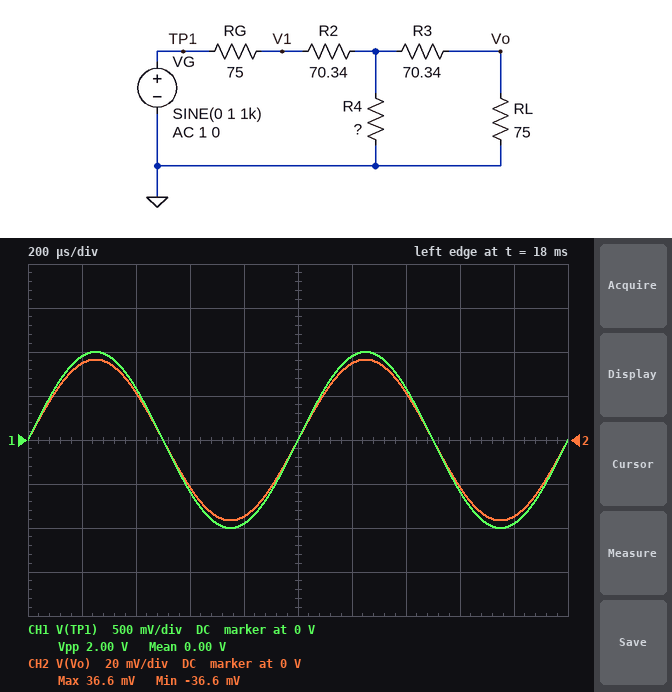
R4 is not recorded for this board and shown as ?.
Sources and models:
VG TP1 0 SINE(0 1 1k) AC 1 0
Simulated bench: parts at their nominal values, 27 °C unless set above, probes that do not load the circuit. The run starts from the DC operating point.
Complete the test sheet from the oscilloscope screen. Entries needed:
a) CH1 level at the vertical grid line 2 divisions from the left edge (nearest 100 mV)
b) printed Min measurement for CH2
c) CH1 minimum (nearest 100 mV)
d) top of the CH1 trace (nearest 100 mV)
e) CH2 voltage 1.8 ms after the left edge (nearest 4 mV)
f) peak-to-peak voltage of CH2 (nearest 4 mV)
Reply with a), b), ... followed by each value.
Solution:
a) 600 mV
b) -36.6 mV
c) -1.0 V
d) 1.0 V
e) -36 mV
f) 72 mV
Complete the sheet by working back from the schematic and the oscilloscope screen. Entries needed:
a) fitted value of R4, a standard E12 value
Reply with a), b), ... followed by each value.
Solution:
a) 12 Ω
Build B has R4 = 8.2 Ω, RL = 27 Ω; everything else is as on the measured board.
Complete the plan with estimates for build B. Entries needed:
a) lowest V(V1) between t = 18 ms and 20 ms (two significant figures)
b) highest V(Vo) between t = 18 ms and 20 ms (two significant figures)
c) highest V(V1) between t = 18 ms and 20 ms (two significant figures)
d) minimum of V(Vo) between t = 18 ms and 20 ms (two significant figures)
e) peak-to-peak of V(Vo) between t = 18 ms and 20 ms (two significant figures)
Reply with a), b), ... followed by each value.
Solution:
a) -510 mV
b) 14 mV
c) 510 mV
d) -14 mV
e) 27 mV
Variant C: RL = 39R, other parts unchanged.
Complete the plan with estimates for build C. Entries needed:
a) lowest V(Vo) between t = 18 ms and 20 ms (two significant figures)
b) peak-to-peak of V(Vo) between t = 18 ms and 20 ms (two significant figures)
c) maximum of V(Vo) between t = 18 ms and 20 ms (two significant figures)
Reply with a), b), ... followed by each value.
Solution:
a) -25 mV
b) 49 mV
c) 25 mV
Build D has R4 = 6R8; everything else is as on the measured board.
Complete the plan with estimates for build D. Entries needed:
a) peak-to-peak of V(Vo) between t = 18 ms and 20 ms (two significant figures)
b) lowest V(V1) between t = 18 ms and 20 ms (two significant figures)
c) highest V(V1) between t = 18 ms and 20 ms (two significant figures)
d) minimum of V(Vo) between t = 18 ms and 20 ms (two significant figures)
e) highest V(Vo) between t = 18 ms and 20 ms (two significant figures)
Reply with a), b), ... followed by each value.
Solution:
a) 44 mV
b) -510 mV
c) 510 mV
d) -22 mV
e) 22 mV
